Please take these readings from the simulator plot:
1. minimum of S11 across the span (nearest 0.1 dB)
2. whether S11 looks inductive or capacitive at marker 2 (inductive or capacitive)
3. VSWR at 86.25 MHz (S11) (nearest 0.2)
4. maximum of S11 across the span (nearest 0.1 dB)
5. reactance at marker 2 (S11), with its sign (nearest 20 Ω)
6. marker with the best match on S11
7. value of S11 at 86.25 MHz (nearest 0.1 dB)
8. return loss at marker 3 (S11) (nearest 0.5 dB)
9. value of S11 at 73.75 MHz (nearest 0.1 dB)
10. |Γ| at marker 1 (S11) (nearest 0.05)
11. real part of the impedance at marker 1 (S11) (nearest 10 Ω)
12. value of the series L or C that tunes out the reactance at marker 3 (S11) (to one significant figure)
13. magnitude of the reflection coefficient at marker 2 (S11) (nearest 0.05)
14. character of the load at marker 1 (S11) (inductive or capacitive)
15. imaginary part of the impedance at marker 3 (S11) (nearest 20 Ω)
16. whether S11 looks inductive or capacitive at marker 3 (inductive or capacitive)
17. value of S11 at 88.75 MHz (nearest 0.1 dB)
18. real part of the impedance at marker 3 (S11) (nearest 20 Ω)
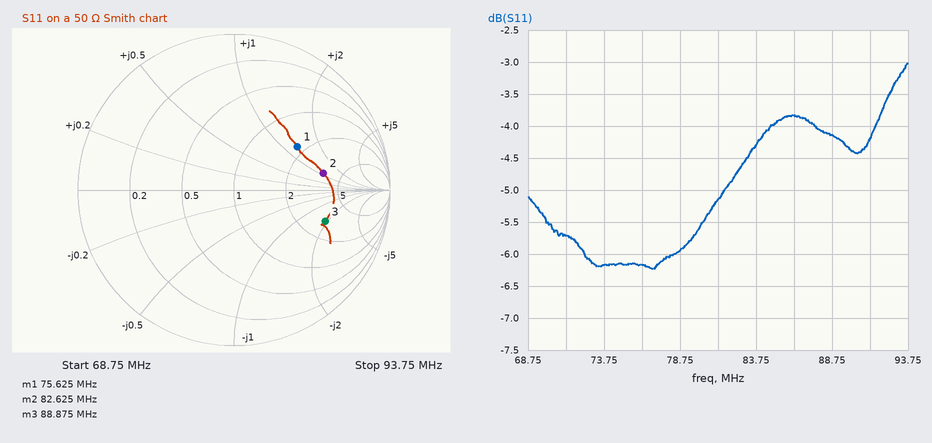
-6.2 dB
inductive
4.6
-3.0 dB
+60 Ω
marker 1
-3.8 dB
4.0 dB
-6.2 dB
0.50
90 Ω
200 nH
0.60
inductive
-100 Ω
capacitive
-4.1 dB
140 Ω
